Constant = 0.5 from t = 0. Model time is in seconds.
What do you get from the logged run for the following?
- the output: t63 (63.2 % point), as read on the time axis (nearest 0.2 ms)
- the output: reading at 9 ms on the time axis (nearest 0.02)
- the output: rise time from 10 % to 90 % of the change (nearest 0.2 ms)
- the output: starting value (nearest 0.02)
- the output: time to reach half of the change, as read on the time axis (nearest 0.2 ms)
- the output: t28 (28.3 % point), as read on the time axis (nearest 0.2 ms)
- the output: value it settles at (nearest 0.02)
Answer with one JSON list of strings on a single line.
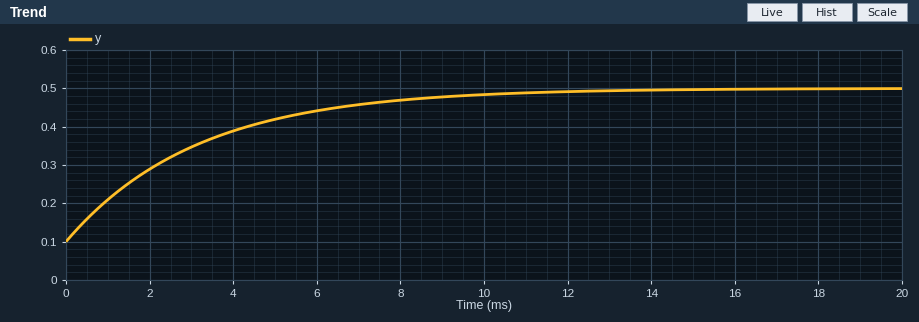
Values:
["3.2 ms", "0.48", "6.8 ms", "0.10", "2.2 ms", "1.0 ms", "0.50"]
